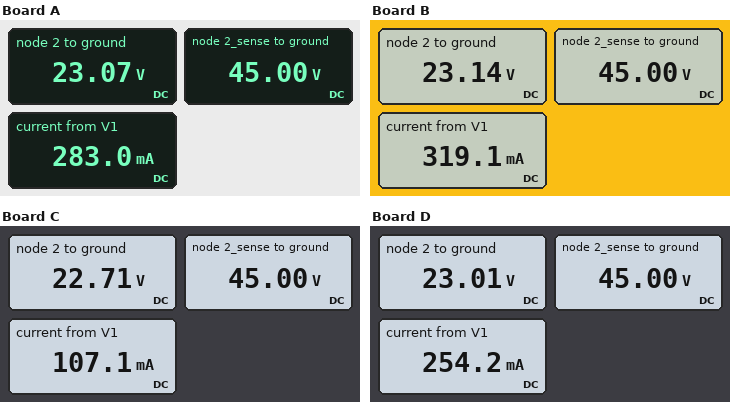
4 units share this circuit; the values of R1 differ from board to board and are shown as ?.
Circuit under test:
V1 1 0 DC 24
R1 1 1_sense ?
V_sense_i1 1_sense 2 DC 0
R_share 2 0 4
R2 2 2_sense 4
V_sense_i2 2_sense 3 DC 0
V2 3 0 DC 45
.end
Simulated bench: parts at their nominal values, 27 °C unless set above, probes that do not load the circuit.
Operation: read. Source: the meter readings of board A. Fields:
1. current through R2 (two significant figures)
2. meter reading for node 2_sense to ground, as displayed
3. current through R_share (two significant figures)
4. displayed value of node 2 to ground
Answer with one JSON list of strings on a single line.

["5.5 A", "45.00 V", "5.8 A", "23.07 V"]
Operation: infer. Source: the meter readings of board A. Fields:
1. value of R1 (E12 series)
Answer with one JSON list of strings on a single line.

["3.3 Ω"]
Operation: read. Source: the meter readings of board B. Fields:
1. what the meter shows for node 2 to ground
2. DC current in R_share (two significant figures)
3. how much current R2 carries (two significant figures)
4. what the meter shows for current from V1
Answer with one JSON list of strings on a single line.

["23.14 V", "5.8 A", "5.5 A", "319.1 mA"]
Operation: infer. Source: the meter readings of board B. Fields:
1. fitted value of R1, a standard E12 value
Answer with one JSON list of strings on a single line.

["2.7 Ω"]
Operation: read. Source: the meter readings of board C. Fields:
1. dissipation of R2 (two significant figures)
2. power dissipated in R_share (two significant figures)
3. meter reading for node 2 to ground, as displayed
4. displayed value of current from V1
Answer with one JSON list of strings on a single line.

["120 W", "130 W", "22.71 V", "107.1 mA"]
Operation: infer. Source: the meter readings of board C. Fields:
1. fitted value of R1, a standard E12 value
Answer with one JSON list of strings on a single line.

["12 Ω"]
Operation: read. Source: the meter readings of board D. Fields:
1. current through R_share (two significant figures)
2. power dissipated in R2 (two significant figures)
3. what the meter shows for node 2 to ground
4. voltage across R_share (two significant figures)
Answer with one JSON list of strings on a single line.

["5.8 A", "120 W", "23.01 V", "23 V"]
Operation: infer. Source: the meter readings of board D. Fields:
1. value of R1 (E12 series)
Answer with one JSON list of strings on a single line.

["3.9 Ω"]
